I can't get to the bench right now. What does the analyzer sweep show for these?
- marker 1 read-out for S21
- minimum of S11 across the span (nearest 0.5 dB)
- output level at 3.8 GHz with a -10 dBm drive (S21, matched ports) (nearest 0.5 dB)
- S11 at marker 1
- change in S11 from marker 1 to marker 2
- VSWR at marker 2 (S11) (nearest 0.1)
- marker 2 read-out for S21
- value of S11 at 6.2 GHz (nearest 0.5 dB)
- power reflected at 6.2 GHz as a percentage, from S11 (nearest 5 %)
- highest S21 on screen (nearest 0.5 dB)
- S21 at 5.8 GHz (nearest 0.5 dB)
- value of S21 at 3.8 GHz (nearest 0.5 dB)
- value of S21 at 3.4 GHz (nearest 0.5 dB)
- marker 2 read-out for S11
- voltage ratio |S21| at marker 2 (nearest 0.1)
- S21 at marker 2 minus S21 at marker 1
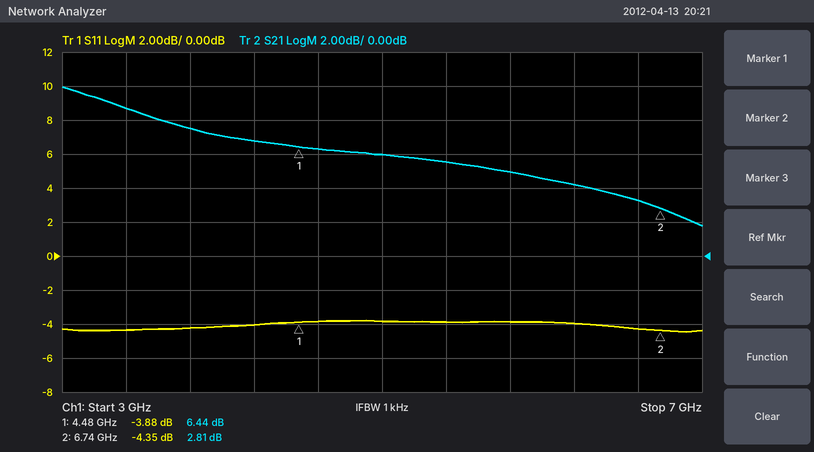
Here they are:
6.44 dB
-4.5 dB
-2.5 dBm
-3.88 dB
-0.47 dB
4.1
2.81 dB
-4.0 dB
40 %
10.0 dB
5.0 dB
7.5 dB
8.5 dB
-4.35 dB
1.4
-3.63 dB
